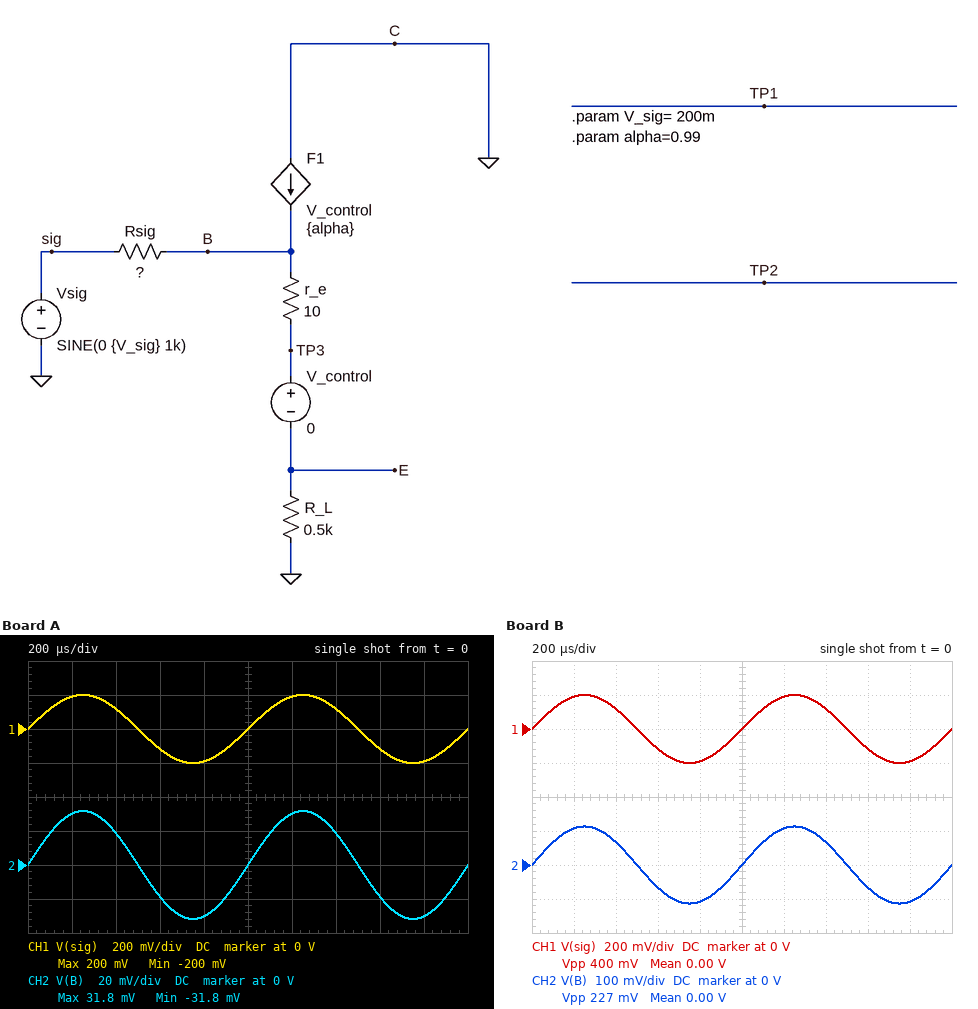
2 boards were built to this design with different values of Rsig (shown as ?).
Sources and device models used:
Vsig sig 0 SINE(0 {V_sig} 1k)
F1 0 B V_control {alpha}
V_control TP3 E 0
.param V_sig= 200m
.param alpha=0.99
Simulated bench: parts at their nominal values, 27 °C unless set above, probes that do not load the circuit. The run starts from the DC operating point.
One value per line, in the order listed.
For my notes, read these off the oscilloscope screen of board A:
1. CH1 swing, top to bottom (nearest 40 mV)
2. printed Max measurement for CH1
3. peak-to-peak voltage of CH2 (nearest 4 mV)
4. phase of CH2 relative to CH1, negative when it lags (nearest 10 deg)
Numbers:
400 mV
200 mV
64 mV
0 deg
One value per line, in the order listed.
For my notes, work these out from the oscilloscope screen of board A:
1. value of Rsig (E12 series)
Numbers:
270 kΩ
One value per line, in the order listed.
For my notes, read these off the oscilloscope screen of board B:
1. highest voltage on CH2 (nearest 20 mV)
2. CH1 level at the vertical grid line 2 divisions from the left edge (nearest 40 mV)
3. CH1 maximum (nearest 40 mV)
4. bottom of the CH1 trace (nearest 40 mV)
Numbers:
120 mV
120 mV
200 mV
-200 mV
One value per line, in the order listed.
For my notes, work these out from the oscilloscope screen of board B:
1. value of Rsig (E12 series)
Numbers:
39 kΩ
